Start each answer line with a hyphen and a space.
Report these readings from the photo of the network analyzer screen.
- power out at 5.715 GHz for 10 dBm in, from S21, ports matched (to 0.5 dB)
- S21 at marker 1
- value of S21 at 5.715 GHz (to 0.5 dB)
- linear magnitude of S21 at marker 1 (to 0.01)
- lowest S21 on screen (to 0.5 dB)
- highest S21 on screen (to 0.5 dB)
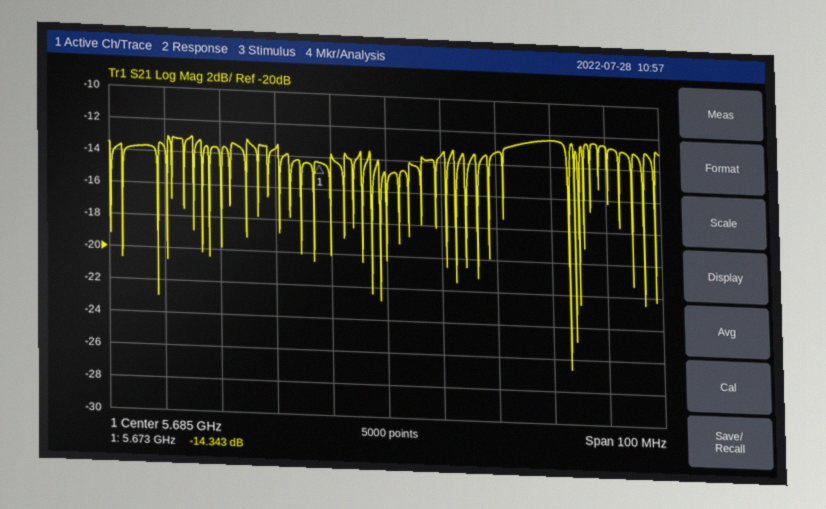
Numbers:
- -2.5 dBm
- -14.343 dB
- -12.5 dB
- 0.19
- -26.5 dB
- -12.5 dB
